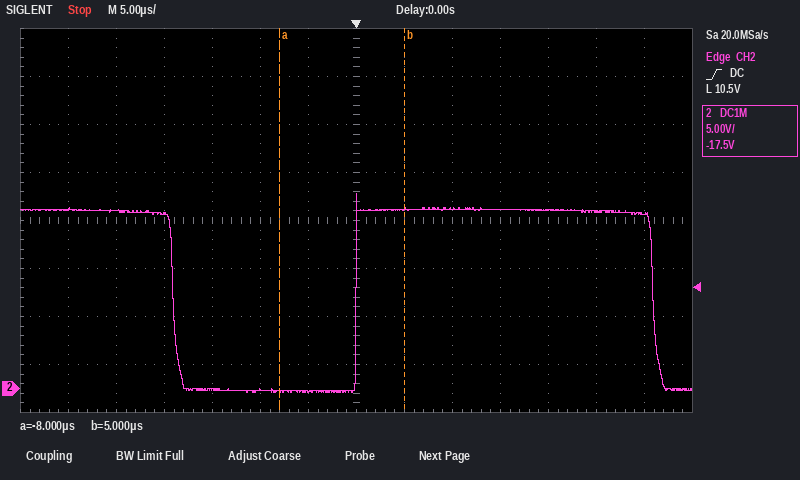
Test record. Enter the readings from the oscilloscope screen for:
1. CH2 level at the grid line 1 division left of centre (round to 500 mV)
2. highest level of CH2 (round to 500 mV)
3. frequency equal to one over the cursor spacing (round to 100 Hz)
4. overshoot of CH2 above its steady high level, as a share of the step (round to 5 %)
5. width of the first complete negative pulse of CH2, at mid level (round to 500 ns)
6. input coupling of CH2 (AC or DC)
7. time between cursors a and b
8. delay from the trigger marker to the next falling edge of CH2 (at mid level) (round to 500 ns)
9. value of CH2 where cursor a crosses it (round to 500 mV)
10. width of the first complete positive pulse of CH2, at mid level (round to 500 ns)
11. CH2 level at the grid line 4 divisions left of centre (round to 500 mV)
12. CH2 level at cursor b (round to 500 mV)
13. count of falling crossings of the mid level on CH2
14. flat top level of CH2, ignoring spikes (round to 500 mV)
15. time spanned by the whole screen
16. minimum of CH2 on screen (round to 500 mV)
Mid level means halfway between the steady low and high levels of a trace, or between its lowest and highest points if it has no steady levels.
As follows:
-500 mV
20.5 V
76.9 kHz
10 %
19.0 µs
DC
13.0 µs
31.0 µs
-500 mV
31.0 µs
18.0 V
18.5 V
2
18.5 V
70 µs
-500 mV
